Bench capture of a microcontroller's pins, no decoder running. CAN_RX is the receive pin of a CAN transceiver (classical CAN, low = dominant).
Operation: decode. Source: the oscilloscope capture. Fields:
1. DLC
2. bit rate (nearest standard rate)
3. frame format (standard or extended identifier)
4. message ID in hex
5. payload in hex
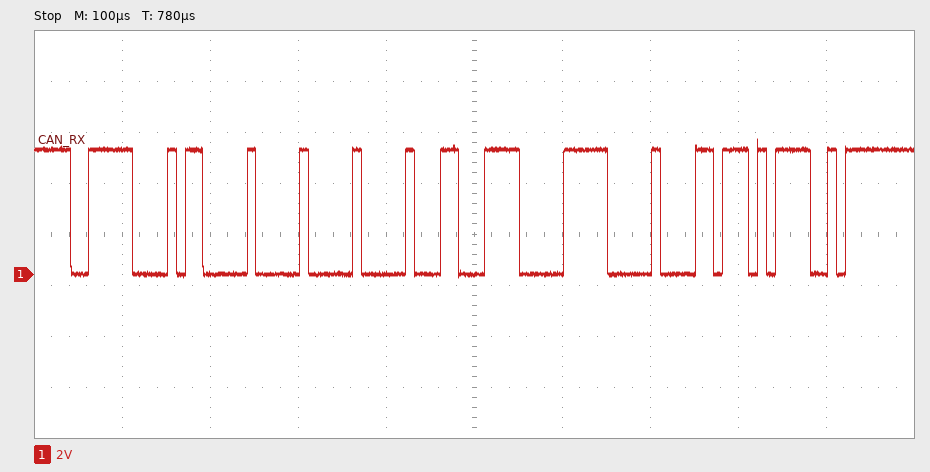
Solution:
3
100 kbit/s
extended
0x0F880000
1E 0F 00
